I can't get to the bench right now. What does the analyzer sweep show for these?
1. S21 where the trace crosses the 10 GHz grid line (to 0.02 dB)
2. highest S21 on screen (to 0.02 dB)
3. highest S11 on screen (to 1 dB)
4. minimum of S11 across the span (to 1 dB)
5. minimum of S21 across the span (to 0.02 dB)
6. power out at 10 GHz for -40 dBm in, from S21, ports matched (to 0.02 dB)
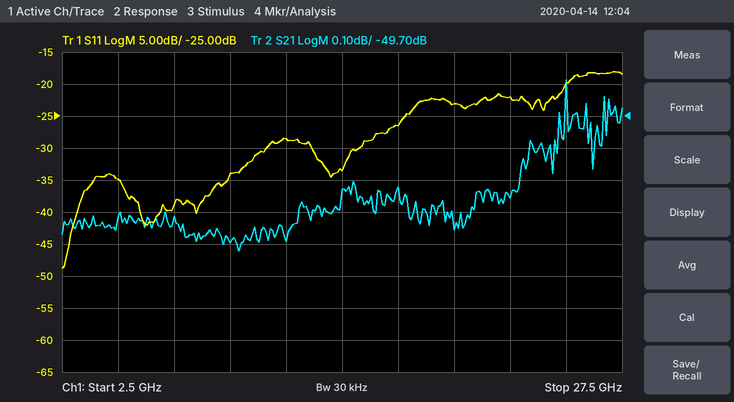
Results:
-50.10 dB
-49.58 dB
-18 dB
-49 dB
-50.12 dB
-90.10 dBm
